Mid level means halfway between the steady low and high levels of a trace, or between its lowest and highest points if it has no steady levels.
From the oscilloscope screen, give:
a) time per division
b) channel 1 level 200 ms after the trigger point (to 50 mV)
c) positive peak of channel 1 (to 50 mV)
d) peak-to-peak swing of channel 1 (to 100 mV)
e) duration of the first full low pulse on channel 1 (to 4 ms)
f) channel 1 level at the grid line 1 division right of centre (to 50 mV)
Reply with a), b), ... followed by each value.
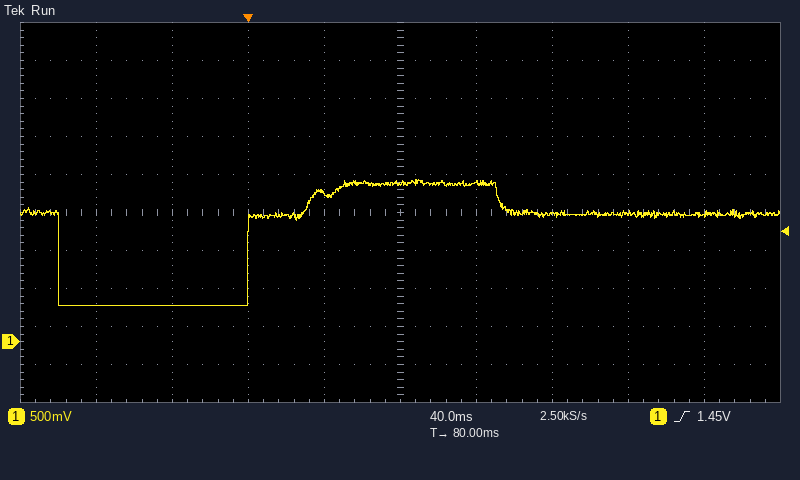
a) 40 ms
b) 1.70 V
c) 2.15 V
d) 1.70 V
e) 100 ms
f) 2.10 V
